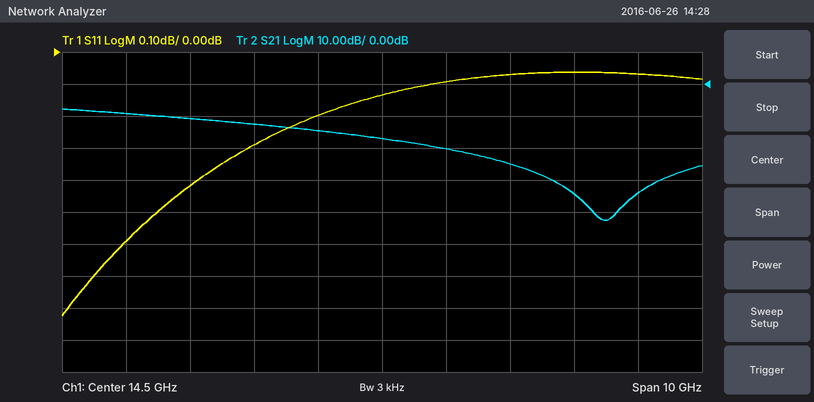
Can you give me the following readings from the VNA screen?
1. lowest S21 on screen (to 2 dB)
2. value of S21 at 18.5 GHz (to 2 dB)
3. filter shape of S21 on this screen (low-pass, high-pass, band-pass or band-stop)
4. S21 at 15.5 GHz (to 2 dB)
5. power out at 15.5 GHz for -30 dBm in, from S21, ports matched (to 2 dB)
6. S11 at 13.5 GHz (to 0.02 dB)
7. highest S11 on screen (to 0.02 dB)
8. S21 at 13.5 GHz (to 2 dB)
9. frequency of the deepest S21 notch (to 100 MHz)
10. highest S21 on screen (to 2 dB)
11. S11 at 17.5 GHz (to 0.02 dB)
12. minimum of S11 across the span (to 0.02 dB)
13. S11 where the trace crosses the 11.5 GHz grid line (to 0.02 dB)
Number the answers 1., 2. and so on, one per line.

1. -42 dB
2. -34 dB
3. low-pass
4. -20 dB
5. -50 dBm
6. -0.20 dB
7. -0.06 dB
8. -14 dB
9. 18.0 GHz
10. -8 dB
11. -0.06 dB
12. -0.82 dB
13. -0.42 dB
